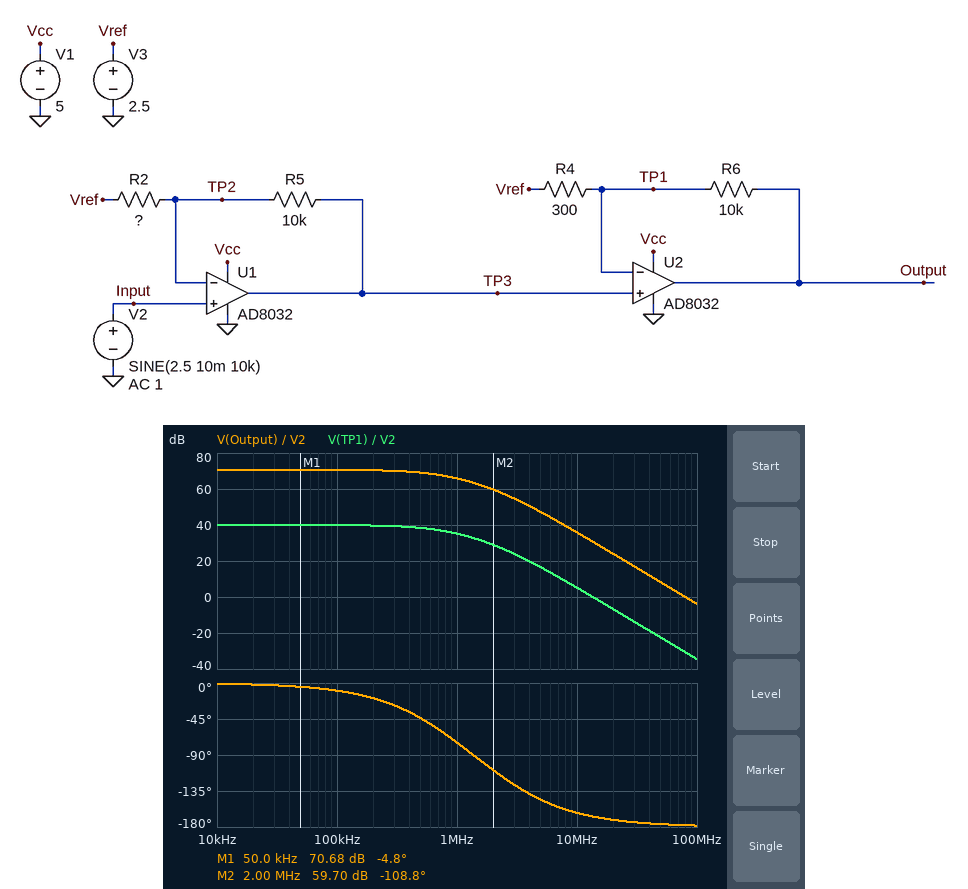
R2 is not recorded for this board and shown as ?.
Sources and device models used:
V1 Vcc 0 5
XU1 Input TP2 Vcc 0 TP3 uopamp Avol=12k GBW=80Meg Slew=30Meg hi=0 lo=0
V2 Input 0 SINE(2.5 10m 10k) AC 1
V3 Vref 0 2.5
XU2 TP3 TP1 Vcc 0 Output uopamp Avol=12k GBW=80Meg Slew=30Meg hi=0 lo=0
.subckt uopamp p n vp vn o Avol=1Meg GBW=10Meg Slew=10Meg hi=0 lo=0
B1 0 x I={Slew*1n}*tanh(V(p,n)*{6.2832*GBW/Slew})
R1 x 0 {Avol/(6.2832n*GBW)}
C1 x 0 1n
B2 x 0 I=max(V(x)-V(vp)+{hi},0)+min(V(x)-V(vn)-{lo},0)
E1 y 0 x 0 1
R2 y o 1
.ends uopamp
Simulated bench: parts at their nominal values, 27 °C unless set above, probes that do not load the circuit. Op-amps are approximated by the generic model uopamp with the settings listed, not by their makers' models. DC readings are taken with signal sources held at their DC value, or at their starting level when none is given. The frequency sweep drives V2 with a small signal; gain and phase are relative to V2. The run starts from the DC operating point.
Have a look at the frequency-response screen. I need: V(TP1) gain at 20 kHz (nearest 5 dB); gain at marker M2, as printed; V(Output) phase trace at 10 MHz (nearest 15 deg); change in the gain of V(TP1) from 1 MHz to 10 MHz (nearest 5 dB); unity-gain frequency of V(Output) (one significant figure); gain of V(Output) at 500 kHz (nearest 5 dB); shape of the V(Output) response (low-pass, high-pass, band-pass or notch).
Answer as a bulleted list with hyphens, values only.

- 40 dB
- 59.70 dB
- -165 deg
- -30 dB
- 80 MHz
- 70 dB
- low-pass
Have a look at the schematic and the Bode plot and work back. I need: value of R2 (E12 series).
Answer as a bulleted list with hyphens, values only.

- 100 Ω
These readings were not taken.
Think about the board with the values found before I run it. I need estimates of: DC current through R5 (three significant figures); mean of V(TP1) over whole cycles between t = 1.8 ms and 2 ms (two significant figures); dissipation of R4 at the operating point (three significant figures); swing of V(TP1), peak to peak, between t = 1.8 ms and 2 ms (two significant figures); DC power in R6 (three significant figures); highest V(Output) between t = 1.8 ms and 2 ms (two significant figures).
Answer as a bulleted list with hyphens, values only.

- 2.07 µA
- 2.5 V
- 1.47 µW
- 150 mV
- 49.1 µW
- 5.0 V
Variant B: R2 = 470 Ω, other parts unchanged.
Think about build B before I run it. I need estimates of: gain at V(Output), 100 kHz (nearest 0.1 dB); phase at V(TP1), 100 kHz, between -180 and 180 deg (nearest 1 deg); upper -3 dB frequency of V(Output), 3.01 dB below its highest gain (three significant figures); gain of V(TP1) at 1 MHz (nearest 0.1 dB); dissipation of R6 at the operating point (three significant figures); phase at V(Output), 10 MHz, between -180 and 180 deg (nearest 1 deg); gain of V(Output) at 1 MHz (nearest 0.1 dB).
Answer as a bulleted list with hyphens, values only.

- 57.6 dB
- -4 deg
- 1.81 MHz
- 25.9 dB
- 2.59 µW
- -147 deg
- 56.6 dB
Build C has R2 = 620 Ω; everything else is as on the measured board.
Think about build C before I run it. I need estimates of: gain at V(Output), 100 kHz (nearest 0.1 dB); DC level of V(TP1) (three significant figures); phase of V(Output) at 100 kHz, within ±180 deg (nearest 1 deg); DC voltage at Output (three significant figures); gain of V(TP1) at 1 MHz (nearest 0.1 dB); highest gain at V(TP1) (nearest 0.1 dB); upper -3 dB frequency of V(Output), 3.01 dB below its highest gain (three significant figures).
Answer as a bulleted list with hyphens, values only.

- 55.3 dB
- 2.50 V
- -4 deg
- 2.37 V
- 23.7 dB
- 24.6 dB
- 1.96 MHz
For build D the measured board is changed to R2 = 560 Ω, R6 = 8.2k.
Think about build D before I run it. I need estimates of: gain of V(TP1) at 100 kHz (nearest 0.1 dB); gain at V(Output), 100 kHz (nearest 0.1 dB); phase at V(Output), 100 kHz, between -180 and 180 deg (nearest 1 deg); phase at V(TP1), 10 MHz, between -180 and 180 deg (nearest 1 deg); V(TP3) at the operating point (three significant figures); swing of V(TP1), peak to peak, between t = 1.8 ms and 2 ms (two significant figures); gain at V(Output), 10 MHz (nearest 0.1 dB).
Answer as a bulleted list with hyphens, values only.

- 25.5 dB
- 54.5 dB
- -3 deg
- -141 deg
- 2.50 V
- 180 mV
- 35.1 dB
